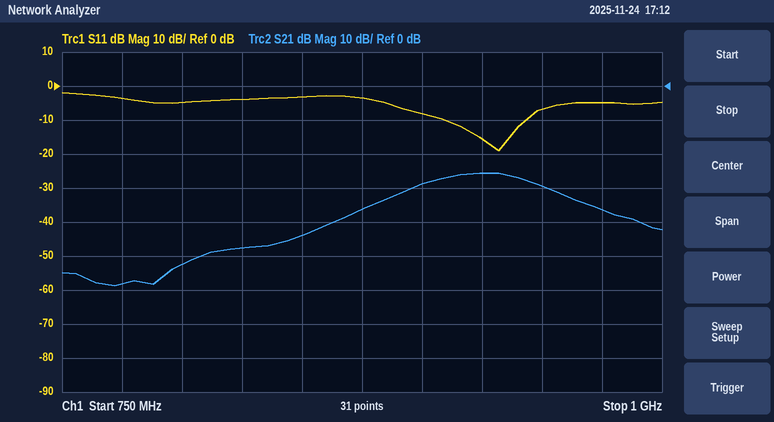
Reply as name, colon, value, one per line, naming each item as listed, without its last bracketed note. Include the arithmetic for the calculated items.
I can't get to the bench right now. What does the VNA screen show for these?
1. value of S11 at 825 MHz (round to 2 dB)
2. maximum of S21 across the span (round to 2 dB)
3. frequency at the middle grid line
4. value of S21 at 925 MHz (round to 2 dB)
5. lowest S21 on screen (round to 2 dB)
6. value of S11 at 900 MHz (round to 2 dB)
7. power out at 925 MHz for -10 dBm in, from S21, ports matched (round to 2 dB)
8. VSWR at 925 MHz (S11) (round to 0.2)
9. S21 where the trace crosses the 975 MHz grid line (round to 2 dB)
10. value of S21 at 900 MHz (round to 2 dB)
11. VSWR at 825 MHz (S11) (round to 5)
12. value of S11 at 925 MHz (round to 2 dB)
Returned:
value of S11 at 825 MHz: -4 dB
maximum of S21 across the span: -26 dB
frequency at the middle grid line: 875 MHz
value of S21 at 925 MHz: -26 dB
lowest S21 on screen: -58 dB
value of S11 at 900 MHz: -8 dB
power out at 925 MHz for -10 dBm in, from S21, ports matched: -10 dBm + (-26 dB) = -36 dBm
VSWR at 925 MHz (S11): |Γ| = 10^(-16/20) = 0.1585; VSWR = (1 + 0.1585)/(1 − 0.1585) ≈ 1.4
S21 where the trace crosses the 975 MHz grid line: -36 dB
value of S21 at 900 MHz: -28 dB
VSWR at 825 MHz (S11): |Γ| = 10^(-4/20) = 0.6310; VSWR = (1 + 0.6310)/(1 − 0.6310) ≈ 4.42, so 5 to the nearest 5
value of S11 at 925 MHz: -16 dB
